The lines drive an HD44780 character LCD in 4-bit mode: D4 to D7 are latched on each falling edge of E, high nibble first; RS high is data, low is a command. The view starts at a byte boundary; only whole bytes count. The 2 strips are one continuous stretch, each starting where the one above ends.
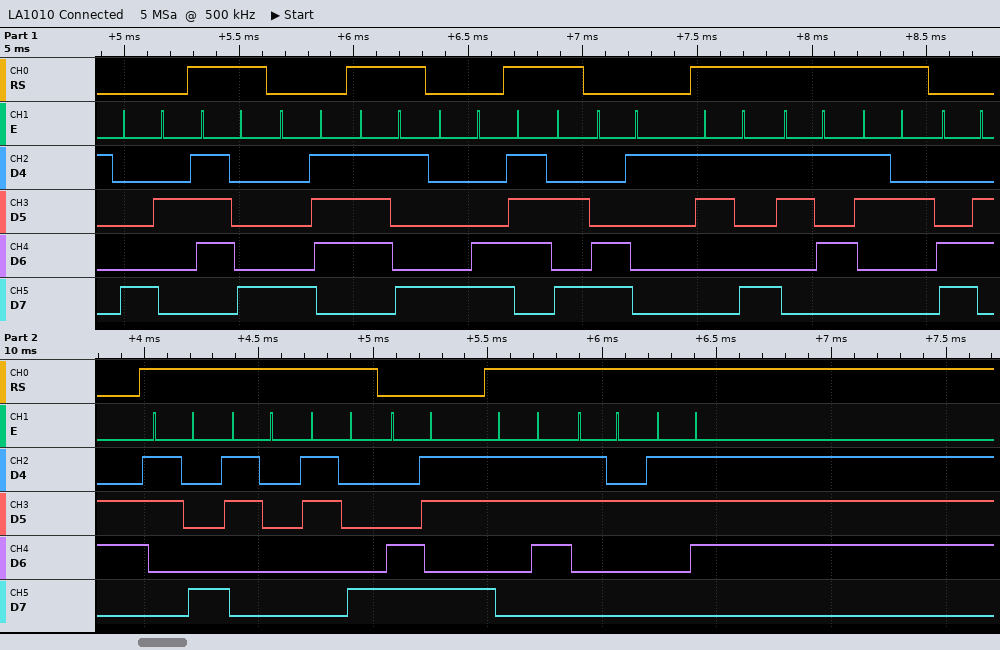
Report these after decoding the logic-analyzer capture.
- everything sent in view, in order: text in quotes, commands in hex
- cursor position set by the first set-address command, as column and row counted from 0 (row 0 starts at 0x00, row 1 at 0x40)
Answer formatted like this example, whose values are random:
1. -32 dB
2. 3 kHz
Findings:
1. 0x82 "x" 0x87 "y" 0x8C "z" 0xC1 "952" 0xC6 "808" 0xCB "727"
2. column 2, row 0
